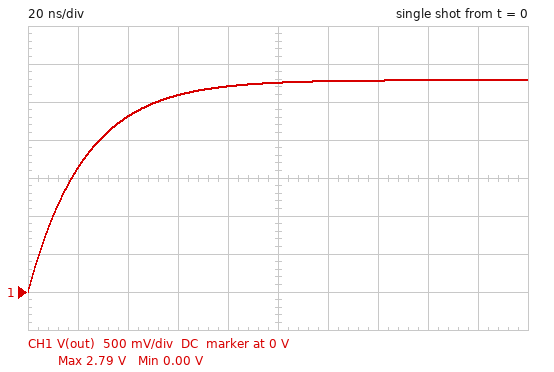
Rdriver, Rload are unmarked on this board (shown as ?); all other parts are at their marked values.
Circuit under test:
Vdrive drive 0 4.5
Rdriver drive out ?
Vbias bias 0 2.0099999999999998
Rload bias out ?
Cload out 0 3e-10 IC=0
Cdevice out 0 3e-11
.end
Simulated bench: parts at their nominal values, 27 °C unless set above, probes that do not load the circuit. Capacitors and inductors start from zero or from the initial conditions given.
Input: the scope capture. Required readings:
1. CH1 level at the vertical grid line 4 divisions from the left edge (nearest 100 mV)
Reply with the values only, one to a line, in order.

2.7 V
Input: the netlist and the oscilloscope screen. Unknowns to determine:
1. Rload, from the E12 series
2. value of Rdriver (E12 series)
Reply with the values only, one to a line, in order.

100 Ω
220 Ω
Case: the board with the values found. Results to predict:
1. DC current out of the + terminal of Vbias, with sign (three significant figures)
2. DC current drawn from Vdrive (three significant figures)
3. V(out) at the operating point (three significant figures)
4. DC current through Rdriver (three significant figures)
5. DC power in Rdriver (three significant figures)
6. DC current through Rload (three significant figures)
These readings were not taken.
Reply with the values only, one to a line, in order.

-7.78 mA
7.78 mA
2.79 V
7.78 mA
13.3 mW
7.78 mA
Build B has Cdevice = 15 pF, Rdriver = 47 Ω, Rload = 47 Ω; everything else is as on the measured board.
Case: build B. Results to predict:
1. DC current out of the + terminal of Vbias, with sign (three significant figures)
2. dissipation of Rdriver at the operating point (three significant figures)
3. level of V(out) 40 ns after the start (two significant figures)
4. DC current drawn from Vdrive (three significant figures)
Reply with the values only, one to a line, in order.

-26.5 mA
33.0 mW
3.2 V
26.5 mA
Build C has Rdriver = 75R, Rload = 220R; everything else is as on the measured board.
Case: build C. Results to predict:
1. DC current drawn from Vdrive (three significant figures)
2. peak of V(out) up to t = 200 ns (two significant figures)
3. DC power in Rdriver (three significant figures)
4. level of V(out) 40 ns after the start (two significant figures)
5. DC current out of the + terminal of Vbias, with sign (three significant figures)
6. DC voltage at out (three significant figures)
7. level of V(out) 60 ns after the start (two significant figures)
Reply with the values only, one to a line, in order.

8.44 mA
3.9 V
5.34 mW
3.4 V
-8.44 mA
3.87 V
3.7 V
